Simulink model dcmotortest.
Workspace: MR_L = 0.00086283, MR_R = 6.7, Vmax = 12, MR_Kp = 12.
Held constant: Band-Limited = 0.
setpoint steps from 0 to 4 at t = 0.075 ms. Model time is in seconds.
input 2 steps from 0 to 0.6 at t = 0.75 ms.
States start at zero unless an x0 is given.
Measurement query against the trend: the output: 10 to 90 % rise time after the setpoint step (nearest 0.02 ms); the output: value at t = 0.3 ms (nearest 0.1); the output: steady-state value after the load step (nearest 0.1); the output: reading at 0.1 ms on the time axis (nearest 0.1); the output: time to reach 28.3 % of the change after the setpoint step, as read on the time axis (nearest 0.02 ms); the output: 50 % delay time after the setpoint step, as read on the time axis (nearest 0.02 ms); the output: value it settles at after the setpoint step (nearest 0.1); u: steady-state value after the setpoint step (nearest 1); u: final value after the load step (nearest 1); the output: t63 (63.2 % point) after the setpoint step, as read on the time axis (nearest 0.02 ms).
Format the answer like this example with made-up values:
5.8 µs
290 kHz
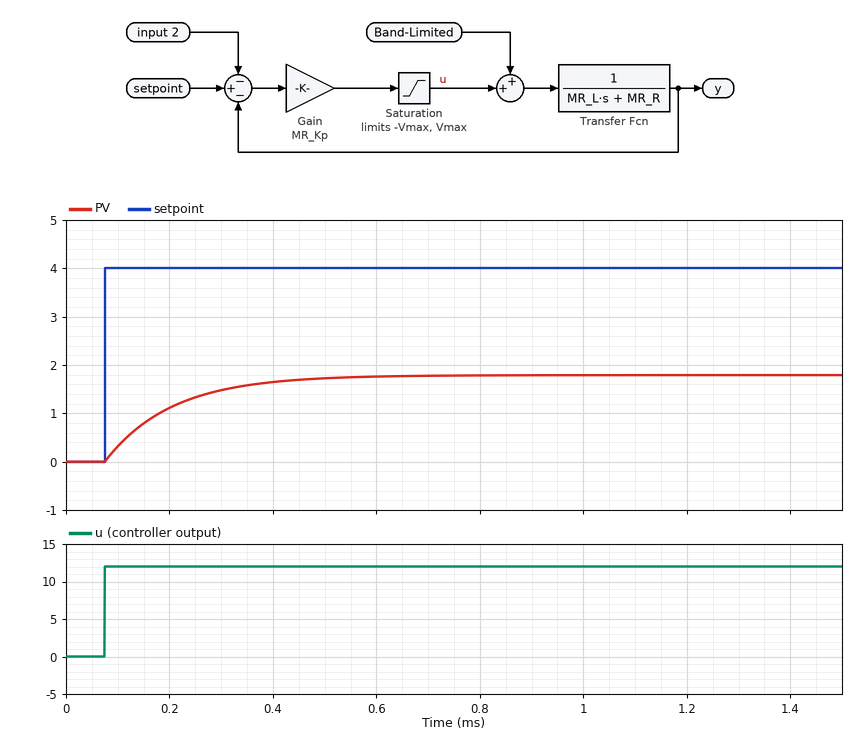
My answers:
0.28 ms
1.5
1.8
0.3
0.12 ms
0.16 ms
1.8
12
12
0.20 ms
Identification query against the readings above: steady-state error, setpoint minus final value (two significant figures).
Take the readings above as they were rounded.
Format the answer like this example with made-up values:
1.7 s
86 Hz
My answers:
2.2
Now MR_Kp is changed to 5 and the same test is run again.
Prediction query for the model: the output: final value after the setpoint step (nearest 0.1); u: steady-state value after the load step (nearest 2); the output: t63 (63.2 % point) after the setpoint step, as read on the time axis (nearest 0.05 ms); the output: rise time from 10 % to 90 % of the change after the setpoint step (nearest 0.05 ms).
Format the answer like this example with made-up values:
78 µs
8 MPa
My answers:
1.7
10
0.20 ms
0.25 ms
